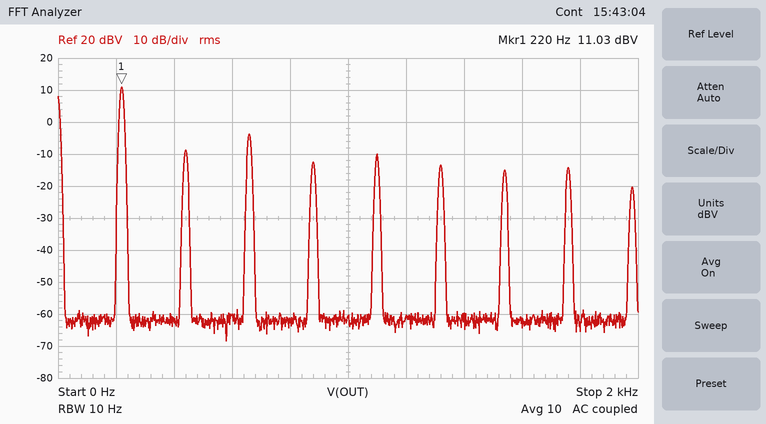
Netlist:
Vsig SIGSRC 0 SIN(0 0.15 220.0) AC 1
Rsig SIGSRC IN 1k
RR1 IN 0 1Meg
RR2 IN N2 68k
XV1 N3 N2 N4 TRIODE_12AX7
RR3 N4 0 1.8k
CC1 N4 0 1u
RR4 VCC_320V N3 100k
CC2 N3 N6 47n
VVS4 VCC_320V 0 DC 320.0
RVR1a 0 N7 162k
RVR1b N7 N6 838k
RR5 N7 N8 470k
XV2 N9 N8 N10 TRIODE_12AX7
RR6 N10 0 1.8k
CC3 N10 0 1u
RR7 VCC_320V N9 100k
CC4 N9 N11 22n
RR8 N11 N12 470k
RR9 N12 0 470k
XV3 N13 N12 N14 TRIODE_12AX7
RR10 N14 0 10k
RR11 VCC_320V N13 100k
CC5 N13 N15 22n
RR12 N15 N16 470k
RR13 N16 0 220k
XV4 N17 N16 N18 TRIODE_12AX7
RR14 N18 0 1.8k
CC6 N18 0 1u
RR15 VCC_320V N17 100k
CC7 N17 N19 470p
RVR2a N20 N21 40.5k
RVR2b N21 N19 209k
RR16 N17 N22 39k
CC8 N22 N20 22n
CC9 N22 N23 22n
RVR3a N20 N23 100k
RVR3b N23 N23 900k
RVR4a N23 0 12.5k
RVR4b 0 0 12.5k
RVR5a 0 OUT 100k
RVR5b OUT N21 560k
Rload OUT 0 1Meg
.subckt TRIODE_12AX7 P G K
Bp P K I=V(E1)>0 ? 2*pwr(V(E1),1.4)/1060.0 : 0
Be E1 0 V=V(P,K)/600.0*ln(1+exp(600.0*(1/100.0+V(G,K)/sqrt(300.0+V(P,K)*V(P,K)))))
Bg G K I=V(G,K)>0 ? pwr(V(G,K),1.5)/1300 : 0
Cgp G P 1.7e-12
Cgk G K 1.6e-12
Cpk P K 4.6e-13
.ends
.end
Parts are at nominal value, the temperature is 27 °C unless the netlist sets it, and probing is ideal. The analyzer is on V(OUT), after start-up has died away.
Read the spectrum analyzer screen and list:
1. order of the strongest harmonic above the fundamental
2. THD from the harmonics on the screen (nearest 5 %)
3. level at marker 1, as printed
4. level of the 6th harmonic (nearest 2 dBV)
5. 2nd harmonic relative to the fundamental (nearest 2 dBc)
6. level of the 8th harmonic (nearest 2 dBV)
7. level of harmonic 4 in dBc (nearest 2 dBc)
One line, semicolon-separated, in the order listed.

3; 25 %; 11.03 dBV; -14 dBV; -20 dBc; -14 dBV; -24 dBc
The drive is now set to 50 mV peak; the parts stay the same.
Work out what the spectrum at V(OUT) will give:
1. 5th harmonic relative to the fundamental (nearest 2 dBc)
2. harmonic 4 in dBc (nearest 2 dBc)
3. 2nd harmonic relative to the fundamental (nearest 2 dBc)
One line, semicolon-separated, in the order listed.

-20 dBc; -36 dBc; -28 dBc
